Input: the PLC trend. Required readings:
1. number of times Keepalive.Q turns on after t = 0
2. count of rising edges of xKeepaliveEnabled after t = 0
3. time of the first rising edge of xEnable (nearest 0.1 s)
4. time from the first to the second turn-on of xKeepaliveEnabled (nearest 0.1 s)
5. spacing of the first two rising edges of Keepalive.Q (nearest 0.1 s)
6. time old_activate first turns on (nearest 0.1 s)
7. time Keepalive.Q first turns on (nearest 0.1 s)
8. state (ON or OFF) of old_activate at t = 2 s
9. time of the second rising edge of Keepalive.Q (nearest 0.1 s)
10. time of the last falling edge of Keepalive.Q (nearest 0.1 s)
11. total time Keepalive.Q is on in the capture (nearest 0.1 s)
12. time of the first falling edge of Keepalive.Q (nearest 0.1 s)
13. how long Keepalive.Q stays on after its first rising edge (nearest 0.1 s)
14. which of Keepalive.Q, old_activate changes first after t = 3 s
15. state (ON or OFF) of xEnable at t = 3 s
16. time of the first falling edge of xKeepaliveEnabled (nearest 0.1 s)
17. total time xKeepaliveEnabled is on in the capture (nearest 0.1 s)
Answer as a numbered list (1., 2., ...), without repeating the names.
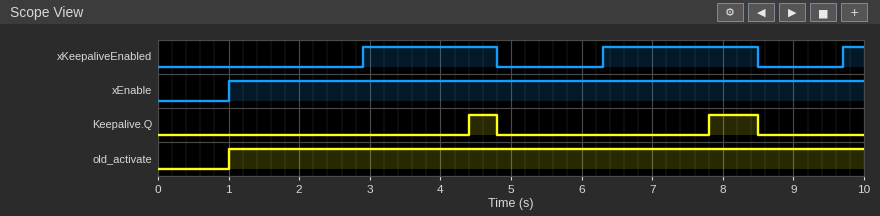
1. 2
2. 3
3. 1.0 s
4. 3.4 s
5. 3.4 s
6. 1.0 s
7. 4.4 s
8. ON
9. 7.8 s
10. 8.5 s
11. 1.1 s
12. 4.8 s
13. 0.4 s
14. Keepalive.Q
15. ON
16. 4.8 s
17. 4.4 s
